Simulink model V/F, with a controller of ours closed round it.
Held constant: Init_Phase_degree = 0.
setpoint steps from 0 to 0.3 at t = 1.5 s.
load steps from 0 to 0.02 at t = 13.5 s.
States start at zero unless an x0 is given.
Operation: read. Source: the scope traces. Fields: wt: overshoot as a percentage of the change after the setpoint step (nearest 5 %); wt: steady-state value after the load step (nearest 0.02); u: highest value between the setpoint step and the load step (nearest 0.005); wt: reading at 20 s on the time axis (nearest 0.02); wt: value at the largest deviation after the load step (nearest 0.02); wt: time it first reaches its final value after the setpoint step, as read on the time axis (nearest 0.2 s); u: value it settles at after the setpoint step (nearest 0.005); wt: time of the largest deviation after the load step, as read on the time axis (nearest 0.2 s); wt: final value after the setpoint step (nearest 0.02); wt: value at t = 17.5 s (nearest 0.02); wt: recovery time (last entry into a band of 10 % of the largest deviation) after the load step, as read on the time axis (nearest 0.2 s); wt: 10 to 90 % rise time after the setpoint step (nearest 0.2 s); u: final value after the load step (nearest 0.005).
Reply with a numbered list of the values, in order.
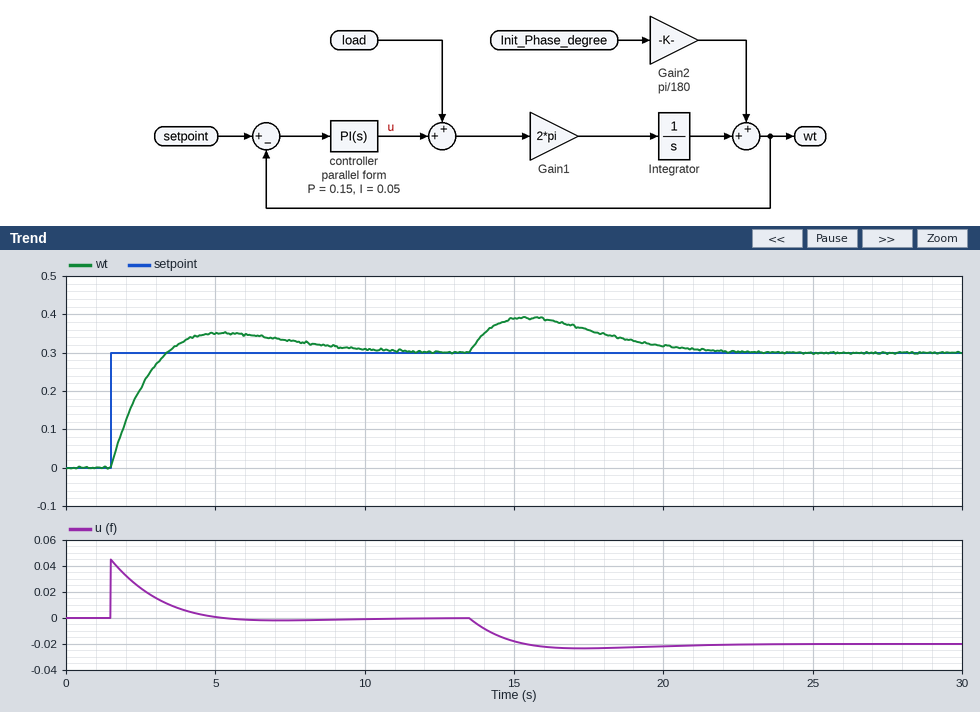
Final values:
1. 15 %
2. 0.30
3. 0.045
4. 0.32
5. 0.40
6. 3.4 s
7. 0.000
8. 15.4 s
9. 0.30
10. 0.36
11. 21.0 s
12. 1.4 s
13. -0.020
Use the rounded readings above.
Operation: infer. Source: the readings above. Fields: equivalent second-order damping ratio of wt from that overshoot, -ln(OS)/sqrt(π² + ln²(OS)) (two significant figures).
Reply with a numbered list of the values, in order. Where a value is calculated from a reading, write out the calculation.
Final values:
1. ln(0.15) = -1.897; 1.897 / sqrt(9.870 + 3.599) = 0.52
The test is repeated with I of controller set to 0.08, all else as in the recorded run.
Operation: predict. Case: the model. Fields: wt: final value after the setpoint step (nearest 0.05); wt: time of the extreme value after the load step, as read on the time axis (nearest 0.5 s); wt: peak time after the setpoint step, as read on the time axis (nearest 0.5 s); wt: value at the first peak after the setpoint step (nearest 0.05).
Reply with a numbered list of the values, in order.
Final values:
1. 0.30
2. 15.0 s
3. 4.5 s
4. 0.35
